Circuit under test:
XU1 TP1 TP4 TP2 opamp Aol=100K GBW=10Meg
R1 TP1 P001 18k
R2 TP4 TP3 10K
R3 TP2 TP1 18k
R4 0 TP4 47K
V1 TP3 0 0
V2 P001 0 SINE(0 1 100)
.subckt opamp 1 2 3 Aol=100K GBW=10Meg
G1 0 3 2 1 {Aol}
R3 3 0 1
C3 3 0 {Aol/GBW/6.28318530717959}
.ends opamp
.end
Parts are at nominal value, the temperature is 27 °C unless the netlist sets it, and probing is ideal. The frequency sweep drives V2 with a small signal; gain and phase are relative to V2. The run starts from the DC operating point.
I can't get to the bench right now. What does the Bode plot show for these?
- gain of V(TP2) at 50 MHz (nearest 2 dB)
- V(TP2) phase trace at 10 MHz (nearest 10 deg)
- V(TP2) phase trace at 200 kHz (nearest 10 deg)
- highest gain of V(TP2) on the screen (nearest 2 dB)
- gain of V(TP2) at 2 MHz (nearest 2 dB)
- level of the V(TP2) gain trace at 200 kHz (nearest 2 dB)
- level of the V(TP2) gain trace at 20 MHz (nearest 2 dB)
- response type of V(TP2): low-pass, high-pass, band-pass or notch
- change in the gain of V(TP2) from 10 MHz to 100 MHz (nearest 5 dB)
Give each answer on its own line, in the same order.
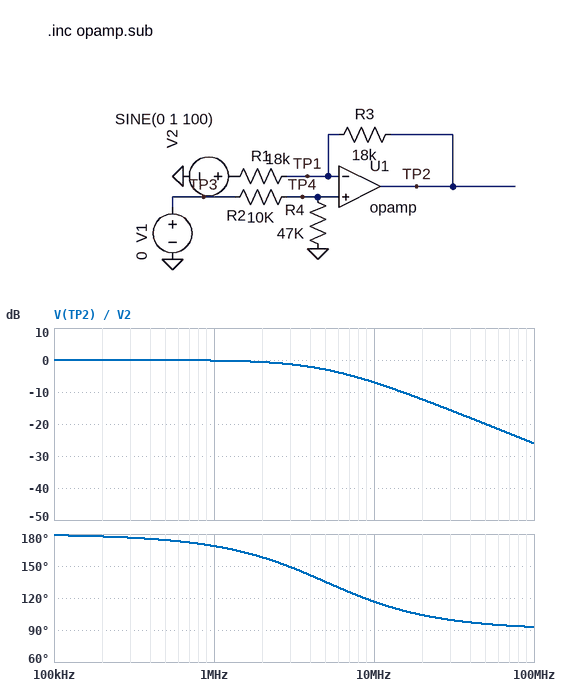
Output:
-20 dB
120 deg
180 deg
0 dB
0 dB
0 dB
-12 dB
low-pass
-20 dB
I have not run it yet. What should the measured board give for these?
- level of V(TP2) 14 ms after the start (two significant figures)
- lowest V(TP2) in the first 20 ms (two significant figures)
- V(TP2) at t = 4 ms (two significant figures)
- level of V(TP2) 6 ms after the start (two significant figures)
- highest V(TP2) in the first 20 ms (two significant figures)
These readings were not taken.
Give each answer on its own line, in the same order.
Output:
-590 mV
-1.0 V
-590 mV
590 mV
1.0 V
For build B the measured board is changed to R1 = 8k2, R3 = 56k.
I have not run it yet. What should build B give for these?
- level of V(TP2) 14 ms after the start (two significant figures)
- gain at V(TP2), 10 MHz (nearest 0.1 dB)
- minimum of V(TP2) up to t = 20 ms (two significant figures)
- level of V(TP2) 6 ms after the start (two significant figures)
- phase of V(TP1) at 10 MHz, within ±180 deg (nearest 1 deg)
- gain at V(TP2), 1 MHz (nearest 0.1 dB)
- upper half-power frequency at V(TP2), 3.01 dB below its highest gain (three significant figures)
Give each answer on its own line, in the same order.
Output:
-4.0 V
-1.3 dB
-6.8 V
4.0 V
7 deg
14.6 dB
1.28 MHz
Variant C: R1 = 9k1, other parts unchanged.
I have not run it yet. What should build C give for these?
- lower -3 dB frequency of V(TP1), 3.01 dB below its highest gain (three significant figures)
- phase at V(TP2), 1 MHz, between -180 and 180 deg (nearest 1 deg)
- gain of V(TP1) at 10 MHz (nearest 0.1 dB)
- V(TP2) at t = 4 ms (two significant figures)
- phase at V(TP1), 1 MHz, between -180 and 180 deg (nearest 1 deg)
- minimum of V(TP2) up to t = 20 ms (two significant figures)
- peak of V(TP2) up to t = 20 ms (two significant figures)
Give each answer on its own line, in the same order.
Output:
3.36 MHz
163 deg
-4.0 dB
-1.2 V
73 deg
-2.0 V
2.0 V
